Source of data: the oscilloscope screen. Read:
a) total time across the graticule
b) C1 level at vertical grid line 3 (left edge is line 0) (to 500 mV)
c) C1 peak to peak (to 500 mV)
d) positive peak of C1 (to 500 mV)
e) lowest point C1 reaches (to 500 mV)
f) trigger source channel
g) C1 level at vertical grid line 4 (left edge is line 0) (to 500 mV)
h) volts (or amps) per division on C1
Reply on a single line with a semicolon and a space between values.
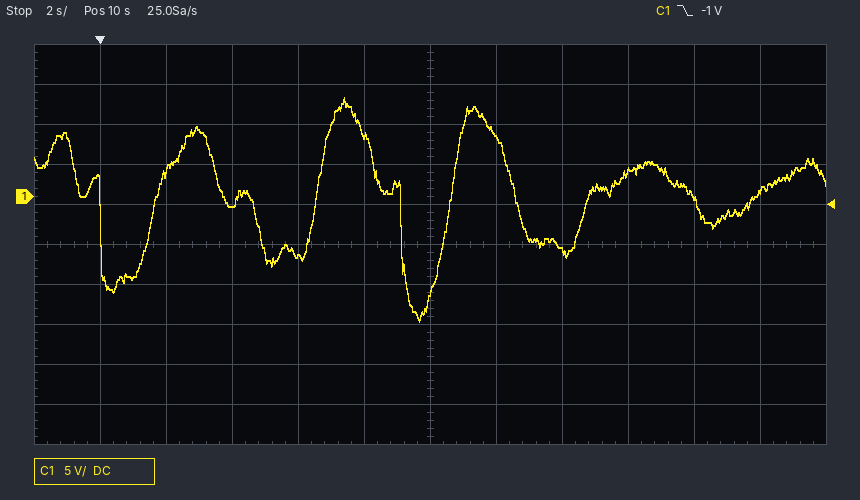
24 s; -1.0 V; 28.0 V; 12.5 V; -15.5 V; C1; -7.5 V; 5 V
